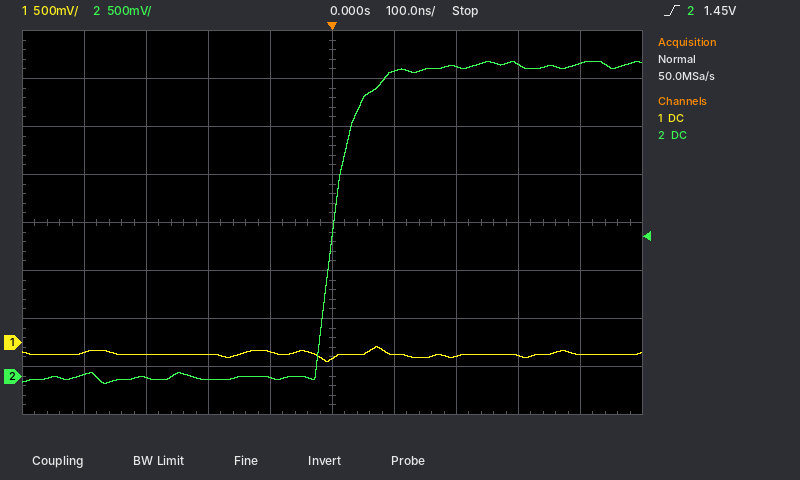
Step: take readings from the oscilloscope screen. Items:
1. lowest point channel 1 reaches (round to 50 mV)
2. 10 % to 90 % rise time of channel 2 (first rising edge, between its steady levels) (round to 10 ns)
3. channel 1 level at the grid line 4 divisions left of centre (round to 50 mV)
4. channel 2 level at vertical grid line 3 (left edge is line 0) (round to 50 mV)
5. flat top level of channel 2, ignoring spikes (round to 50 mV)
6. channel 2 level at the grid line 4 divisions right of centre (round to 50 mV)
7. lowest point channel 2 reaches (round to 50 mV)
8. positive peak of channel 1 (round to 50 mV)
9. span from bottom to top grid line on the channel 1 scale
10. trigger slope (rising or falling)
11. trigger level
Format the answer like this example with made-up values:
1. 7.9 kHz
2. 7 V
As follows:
1. -200 mV
2. 70 ns
3. -100 mV
4. -50 mV
5. 3.20 V
6. 3.25 V
7. -100 mV
8. -50 mV
9. 4 V
10. rising
11. 1.45 V
